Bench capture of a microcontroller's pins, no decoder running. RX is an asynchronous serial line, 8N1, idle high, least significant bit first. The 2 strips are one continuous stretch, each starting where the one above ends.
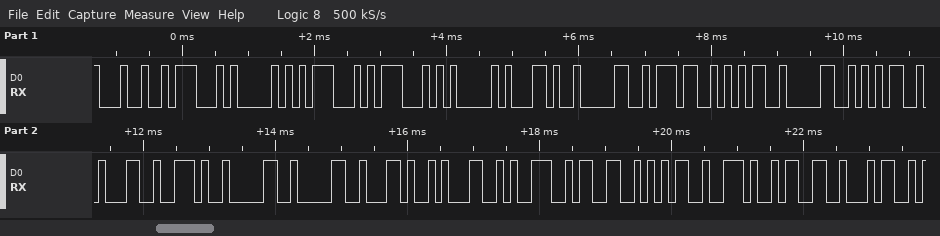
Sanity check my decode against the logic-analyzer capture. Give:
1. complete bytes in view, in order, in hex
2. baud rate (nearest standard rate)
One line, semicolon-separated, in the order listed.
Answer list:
24 47 50 47 47 41 2C 30 37 35 30 35 31 2E 30 30 2C 31 39 33 35 2E 33 34; 9600 baud
